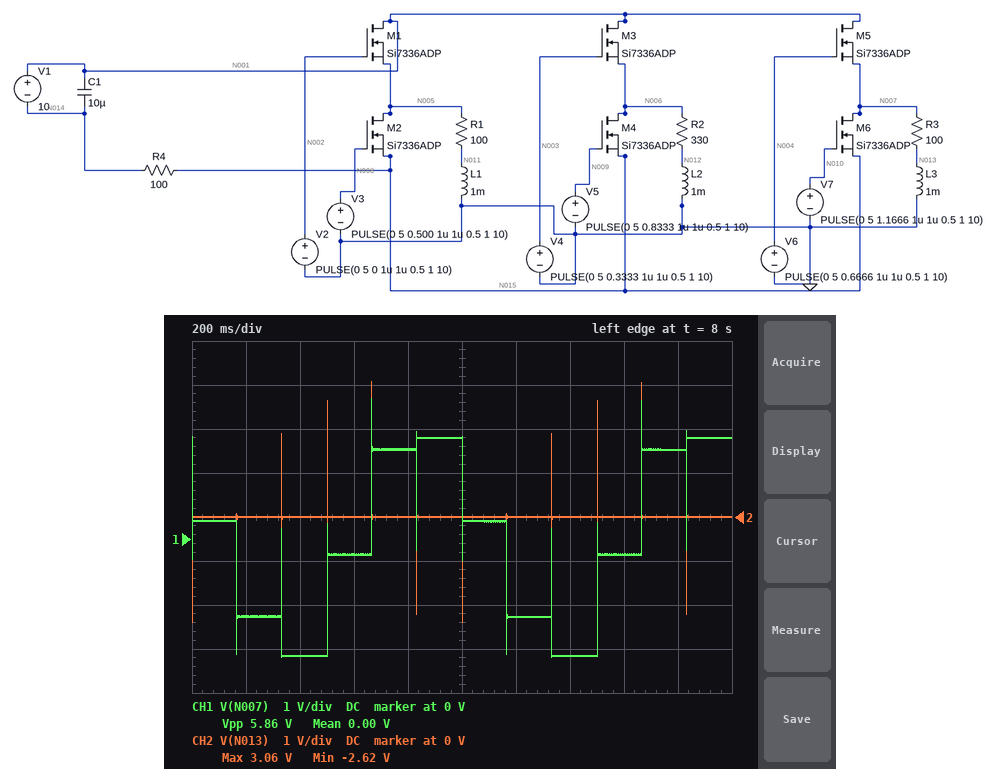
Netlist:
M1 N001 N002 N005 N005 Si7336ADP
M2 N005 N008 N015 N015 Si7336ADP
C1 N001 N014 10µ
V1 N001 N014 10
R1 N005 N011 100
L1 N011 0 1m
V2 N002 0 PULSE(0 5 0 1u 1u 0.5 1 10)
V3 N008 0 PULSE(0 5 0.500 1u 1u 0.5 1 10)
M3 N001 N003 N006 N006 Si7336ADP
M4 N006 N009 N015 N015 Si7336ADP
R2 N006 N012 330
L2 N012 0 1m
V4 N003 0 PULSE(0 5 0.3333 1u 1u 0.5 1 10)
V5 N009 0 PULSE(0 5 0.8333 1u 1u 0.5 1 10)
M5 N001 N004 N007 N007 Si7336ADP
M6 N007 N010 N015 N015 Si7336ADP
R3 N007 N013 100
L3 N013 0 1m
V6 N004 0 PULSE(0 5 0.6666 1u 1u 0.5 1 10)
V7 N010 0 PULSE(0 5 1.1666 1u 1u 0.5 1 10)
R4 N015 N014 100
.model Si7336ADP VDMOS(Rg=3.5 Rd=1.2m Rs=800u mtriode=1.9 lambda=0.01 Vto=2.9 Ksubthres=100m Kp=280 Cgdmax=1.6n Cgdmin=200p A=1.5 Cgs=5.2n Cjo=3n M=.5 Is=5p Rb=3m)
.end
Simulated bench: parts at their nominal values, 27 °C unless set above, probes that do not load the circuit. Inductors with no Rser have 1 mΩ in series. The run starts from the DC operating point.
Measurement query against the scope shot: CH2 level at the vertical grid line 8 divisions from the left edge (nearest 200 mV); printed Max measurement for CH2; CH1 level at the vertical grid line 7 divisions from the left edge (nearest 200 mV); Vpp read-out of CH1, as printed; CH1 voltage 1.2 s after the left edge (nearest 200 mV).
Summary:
0 V
3.06 V
-2.6 V
5.86 V
-1.8 V
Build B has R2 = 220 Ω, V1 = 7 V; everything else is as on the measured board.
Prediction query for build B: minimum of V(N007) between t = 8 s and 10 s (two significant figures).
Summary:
-2.6 V
